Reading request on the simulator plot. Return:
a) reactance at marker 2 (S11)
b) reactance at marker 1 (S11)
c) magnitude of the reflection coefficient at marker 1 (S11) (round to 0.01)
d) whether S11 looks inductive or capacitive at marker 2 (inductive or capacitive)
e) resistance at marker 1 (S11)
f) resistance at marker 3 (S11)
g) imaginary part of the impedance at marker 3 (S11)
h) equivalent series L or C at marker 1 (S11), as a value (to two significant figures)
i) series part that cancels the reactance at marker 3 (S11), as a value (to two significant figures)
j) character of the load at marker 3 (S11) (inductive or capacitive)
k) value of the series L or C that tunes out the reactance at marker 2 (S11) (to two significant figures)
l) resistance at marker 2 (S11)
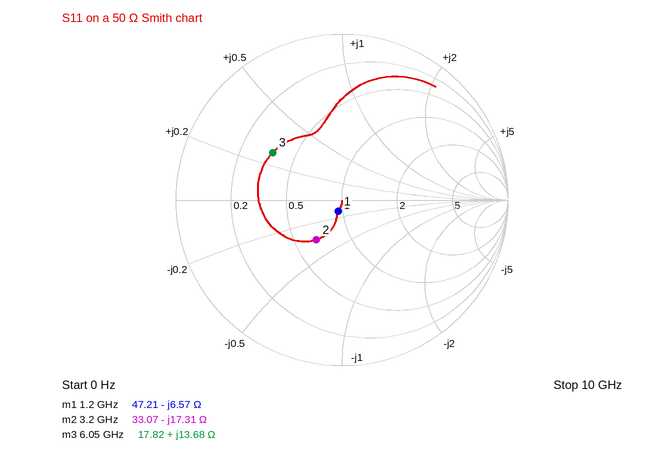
-17.31 Ω
-6.57 Ω
0.07
capacitive
47.21 Ω
17.82 Ω
+13.68 Ω
20 pF
1.9 pF
inductive
860 pH
33.07 Ω
